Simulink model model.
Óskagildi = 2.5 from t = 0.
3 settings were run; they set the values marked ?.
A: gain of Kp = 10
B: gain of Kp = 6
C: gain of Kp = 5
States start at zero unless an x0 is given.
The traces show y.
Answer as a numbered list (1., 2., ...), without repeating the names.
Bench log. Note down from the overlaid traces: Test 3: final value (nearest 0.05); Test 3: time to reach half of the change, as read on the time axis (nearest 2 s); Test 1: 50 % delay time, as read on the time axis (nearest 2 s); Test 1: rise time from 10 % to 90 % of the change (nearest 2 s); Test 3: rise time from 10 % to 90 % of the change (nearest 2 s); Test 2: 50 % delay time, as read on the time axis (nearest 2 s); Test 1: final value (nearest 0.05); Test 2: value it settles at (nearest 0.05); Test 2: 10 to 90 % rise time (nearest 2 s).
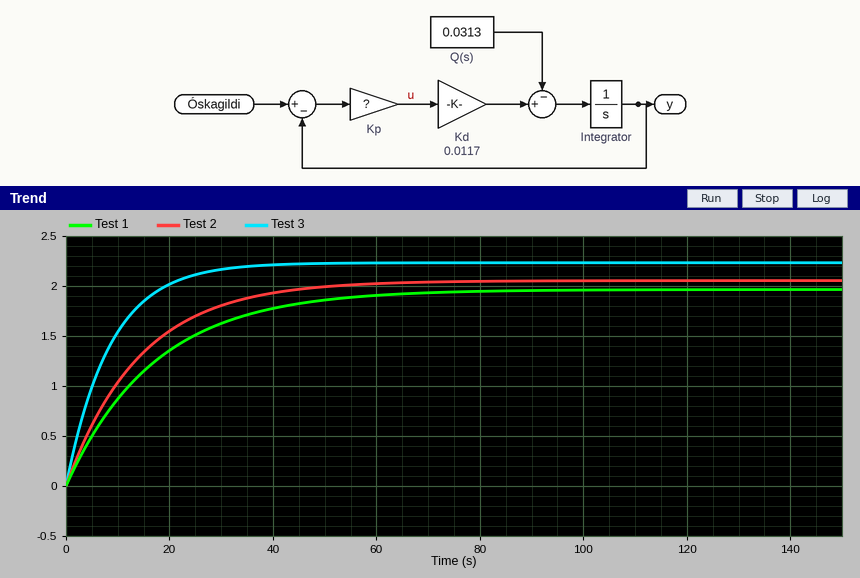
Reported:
1. 2.25
2. 6 s
3. 12 s
4. 38 s
5. 18 s
6. 10 s
7. 1.95
8. 2.05
9. 32 s
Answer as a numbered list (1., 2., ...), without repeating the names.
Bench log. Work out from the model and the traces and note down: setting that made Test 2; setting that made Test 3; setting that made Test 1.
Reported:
1. B
2. A
3. C
